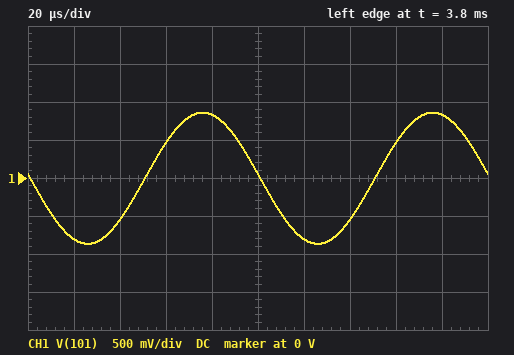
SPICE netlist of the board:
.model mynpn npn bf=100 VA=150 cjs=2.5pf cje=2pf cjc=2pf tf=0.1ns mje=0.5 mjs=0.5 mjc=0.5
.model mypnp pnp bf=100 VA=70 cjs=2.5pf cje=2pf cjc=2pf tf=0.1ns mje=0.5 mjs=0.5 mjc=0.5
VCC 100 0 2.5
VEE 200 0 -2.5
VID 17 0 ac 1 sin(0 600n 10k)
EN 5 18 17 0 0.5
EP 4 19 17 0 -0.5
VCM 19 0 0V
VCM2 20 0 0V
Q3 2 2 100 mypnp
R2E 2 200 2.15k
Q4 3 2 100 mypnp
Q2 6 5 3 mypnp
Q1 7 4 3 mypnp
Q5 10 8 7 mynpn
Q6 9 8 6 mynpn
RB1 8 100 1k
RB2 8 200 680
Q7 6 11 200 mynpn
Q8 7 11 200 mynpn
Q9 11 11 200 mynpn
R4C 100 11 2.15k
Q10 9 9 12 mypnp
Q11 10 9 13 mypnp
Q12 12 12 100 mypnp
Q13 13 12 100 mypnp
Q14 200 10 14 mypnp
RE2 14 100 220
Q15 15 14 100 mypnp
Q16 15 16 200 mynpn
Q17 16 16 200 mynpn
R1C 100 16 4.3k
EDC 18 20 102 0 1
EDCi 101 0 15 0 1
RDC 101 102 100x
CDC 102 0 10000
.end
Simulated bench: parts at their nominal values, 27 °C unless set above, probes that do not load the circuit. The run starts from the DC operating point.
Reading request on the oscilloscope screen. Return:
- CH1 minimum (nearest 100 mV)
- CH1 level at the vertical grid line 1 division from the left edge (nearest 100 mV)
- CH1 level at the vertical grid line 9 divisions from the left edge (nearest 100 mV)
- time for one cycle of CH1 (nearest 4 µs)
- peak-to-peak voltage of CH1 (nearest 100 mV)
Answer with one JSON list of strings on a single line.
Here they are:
["-900 mV", "-800 mV", "800 mV", "100 µs", "1.7 V"]
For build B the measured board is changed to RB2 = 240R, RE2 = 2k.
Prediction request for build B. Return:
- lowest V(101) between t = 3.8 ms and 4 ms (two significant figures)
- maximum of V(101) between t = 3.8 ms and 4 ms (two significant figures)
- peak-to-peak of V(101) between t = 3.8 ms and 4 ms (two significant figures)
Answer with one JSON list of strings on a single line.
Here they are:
["-2.4 V", "2.3 V", "4.7 V"]
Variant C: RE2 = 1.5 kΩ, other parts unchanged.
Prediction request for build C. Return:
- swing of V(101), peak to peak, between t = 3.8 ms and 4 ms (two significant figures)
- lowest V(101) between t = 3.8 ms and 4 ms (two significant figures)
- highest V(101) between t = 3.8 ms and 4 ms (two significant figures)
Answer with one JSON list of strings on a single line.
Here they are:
["4.7 V", "-2.4 V", "2.3 V"]
